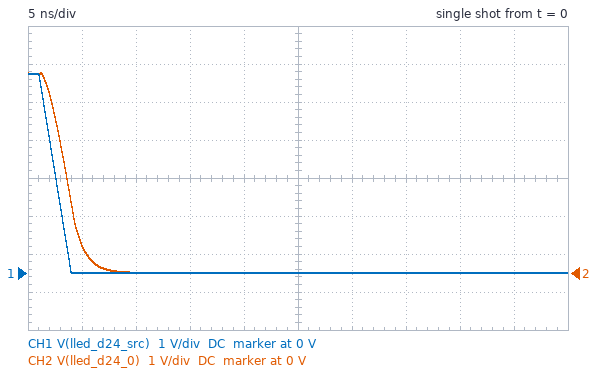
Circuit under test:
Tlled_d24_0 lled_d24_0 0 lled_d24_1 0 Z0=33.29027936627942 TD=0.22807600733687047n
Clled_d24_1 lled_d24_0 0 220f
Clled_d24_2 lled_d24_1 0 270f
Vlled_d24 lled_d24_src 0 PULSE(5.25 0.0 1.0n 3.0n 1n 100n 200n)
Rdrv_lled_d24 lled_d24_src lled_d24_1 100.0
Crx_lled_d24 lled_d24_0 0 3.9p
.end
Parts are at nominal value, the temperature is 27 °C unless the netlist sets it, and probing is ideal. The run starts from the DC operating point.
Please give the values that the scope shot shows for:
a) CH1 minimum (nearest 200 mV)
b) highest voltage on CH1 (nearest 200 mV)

0 V
5.2 V
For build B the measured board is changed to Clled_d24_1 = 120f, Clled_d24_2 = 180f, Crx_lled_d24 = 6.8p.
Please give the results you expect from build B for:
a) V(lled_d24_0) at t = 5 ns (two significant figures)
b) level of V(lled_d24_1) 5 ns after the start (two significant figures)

1.0 V
1.1 V
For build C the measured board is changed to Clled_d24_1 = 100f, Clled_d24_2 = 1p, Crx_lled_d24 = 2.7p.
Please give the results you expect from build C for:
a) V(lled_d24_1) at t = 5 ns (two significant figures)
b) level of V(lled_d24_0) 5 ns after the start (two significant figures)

700 mV
650 mV
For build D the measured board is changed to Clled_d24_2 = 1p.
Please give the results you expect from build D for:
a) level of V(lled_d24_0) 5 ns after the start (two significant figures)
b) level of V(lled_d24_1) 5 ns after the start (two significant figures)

800 mV
850 mV
